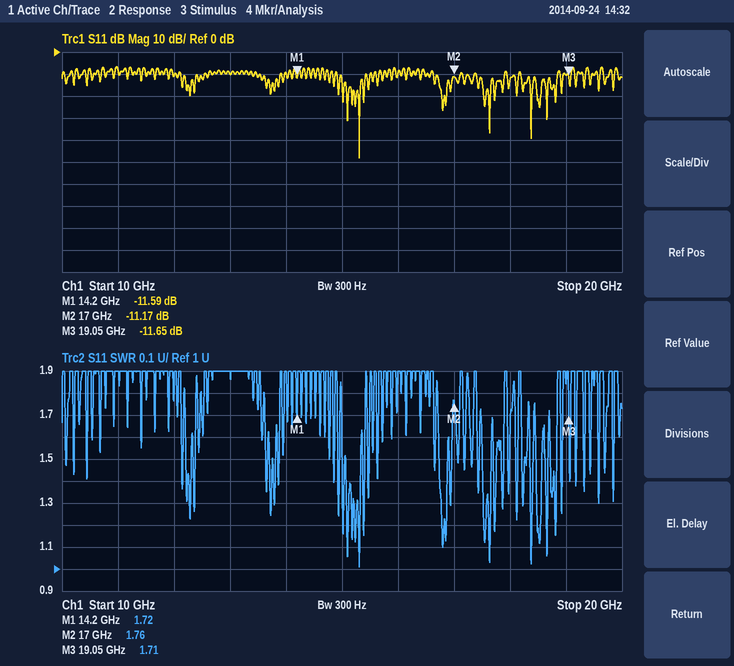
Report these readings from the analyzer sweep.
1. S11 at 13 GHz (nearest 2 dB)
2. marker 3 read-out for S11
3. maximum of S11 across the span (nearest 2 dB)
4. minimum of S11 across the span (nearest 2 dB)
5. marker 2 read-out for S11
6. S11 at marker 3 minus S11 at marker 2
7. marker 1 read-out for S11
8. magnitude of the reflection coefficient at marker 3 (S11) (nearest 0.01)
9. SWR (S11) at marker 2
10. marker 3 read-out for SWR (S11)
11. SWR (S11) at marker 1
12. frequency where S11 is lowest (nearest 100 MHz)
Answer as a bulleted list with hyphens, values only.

- -10 dB
- -11.65 dB
- -6 dB
- -48 dB
- -11.17 dB
- -0.48 dB
- -11.59 dB
- 0.26
- 1.76
- 1.71
- 1.72
- 15.3 GHz
